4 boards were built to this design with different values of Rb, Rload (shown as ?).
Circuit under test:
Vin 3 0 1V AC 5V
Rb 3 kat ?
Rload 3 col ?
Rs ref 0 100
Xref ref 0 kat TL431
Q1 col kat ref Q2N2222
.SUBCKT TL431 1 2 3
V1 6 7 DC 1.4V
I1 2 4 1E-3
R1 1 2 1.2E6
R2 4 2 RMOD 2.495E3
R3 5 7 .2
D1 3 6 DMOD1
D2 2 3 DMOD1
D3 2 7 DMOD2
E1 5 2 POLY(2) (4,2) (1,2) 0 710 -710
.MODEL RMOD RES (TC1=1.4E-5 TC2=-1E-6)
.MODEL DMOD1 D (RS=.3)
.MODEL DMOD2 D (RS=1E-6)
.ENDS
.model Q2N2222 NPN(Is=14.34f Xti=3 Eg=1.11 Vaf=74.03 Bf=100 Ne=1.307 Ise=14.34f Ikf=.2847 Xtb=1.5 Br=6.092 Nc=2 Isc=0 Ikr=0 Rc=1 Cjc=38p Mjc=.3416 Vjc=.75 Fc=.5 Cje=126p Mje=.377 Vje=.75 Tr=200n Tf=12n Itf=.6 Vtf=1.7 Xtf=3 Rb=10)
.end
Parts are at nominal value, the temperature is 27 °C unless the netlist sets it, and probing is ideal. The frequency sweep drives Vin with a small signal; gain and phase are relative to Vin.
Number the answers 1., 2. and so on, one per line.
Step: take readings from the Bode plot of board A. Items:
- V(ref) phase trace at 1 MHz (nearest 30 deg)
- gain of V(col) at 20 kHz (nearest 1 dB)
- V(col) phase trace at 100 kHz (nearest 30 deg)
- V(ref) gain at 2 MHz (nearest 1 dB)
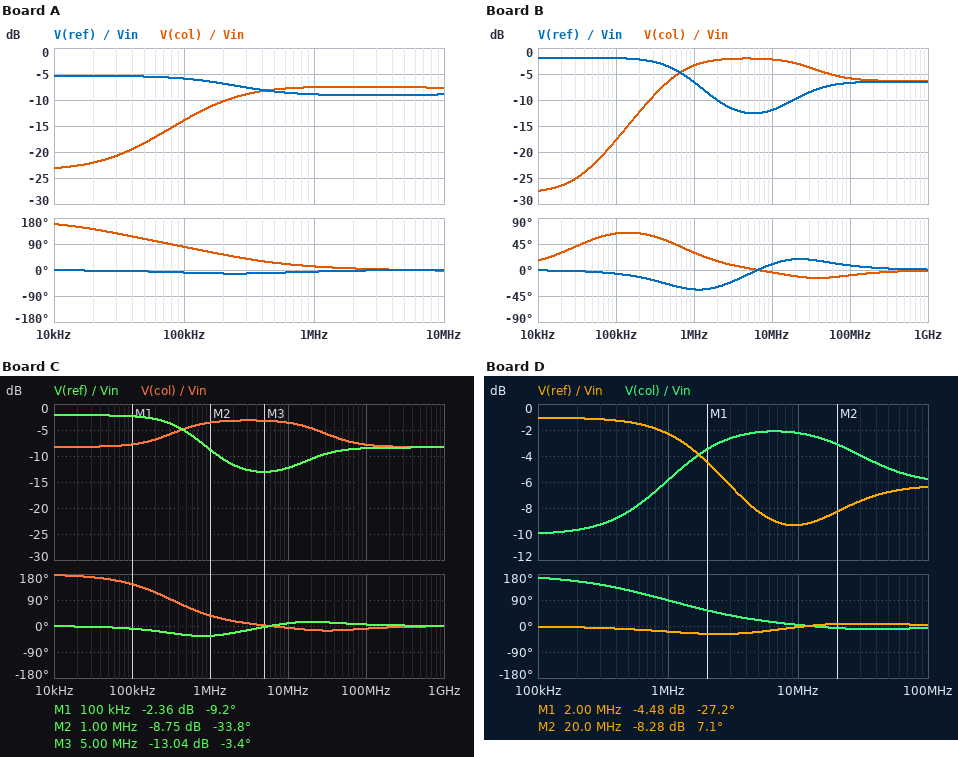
1. 0 deg
2. -22 dB
3. 90 deg
4. -9 dB
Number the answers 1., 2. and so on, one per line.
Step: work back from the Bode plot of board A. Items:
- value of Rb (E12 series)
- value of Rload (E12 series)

1. 680 Ω
2. 220 Ω
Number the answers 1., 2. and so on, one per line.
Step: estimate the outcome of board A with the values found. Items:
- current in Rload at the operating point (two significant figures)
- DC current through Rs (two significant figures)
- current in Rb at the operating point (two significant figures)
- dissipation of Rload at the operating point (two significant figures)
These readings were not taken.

1. 2.8 mA
2. 2.9 mA
3. 54 µA
4. 1.8 mW
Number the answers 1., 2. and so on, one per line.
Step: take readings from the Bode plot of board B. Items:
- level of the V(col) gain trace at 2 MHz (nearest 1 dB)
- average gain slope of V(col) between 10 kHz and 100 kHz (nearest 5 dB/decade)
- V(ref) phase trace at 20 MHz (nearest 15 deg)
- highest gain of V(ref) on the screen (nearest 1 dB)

1. -2 dB
2. 10 dB/decade
3. 15 deg
4. -2 dB
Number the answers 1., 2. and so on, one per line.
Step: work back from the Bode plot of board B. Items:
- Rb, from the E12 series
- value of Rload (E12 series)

1. 1.2 kΩ
2. 120 Ω
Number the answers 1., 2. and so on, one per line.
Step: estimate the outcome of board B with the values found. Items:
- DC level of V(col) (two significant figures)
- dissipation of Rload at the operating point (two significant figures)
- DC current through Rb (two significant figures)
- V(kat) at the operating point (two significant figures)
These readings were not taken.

1. 660 mV
2. 950 µW
3. 35 µA
4. 960 mV
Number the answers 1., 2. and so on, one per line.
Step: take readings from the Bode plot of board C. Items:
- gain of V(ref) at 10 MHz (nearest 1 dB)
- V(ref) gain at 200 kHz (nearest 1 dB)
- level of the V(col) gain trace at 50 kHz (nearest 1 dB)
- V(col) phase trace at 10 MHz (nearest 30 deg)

1. -12 dB
2. -3 dB
3. -8 dB
4. 0 deg
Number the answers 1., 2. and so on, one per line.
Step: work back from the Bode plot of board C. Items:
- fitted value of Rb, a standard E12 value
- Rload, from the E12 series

1. 1.5 kΩ
2. 180 Ω
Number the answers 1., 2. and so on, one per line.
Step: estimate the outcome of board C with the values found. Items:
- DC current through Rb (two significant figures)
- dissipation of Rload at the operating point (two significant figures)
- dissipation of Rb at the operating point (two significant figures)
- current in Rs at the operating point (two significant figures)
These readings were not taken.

1. 34 µA
2. 1.3 mW
3. 1.7 µW
4. 2.8 mA
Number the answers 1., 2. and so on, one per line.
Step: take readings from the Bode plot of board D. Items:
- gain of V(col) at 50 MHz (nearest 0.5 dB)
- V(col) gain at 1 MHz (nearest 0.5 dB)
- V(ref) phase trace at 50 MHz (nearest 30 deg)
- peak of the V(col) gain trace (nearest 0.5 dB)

1. -5.0 dB
2. -6.0 dB
3. 0 deg
4. -2.0 dB
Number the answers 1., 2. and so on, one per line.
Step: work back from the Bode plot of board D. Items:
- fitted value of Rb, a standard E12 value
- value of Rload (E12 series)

1. 330 Ω
2. 150 Ω
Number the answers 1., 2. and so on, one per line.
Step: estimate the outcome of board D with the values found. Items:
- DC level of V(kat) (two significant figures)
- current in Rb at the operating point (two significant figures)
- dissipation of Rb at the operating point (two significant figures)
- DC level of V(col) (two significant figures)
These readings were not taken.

1. 990 mV
2. 38 µA
3. 480 nW
4. 540 mV
